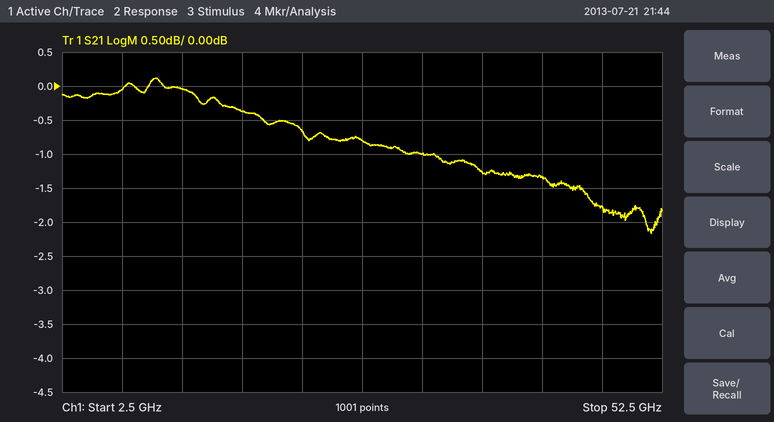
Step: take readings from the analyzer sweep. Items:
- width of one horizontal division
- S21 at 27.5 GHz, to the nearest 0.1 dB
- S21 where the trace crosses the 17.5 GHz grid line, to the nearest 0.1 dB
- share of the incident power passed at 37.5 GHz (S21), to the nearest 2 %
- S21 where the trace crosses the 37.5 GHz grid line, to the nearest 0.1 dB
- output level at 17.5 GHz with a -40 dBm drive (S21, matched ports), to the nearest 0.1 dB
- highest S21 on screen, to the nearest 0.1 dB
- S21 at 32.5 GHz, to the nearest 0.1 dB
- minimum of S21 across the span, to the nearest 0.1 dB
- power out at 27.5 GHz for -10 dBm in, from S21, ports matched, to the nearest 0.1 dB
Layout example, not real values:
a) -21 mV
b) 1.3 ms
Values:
a) 5 GHz
b) -0.8 dB
c) -0.4 dB
d) 74 %
e) -1.3 dB
f) -40.4 dBm
g) 0.1 dB
h) -1.0 dB
i) -2.2 dB
j) -10.8 dBm
